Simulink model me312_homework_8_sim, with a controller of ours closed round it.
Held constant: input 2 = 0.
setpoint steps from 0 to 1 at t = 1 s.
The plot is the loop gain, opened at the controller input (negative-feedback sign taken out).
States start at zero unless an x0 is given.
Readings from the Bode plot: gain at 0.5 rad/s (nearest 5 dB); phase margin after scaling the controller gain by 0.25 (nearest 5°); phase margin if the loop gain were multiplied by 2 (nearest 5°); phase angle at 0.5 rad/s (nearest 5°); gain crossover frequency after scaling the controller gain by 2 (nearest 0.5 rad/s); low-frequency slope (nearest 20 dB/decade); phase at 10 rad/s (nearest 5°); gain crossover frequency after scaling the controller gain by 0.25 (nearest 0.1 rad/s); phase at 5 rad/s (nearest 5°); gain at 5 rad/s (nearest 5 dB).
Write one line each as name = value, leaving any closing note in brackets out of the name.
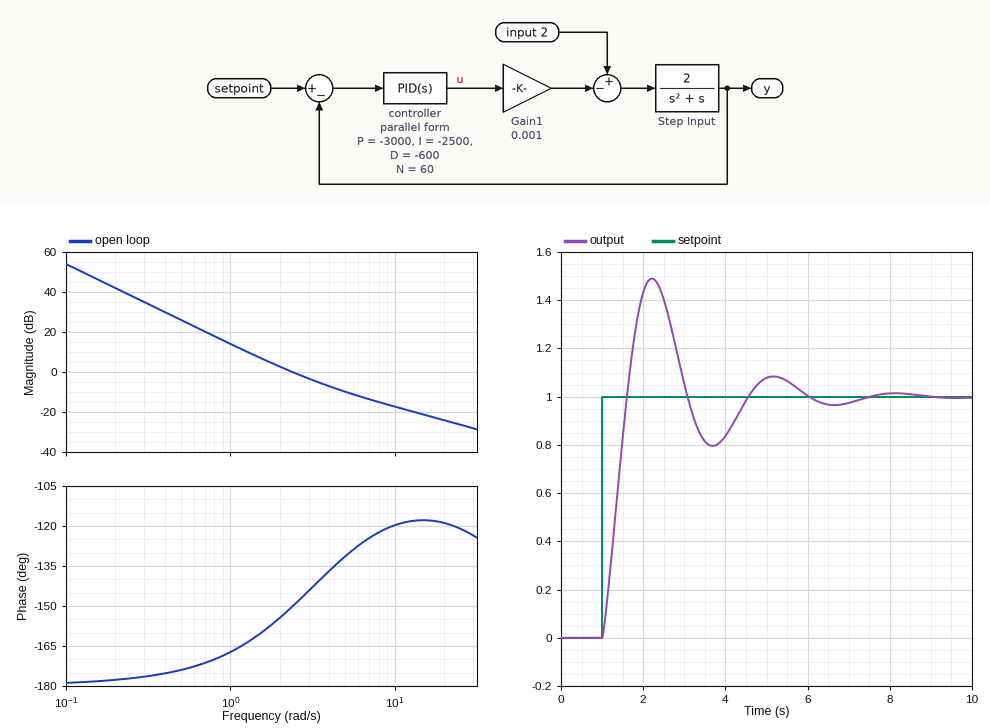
gain at 0.5 rad/s = 25 dB
phase margin after scaling the controller gain by 0.25 = 15°
phase margin if the loop gain were multiplied by 2 = 40°
phase angle at 0.5 rad/s = -175°
gain crossover frequency after scaling the controller gain by 2 = 3.5 rad/s
low-frequency slope = -40 dB/decade
phase at 10 rad/s = -120°
gain crossover frequency after scaling the controller gain by 0.25 = 1.1 rad/s
phase at 5 rad/s = -130°
gain at 5 rad/s = -10 dB
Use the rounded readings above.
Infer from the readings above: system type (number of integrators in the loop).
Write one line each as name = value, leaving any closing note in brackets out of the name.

system type = 2
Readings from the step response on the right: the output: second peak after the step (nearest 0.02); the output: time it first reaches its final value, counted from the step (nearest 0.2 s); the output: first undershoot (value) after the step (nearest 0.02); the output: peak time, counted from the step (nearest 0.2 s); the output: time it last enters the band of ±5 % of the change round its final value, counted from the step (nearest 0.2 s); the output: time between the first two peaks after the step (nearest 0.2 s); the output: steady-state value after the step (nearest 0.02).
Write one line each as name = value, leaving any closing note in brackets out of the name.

the output: second peak after the step = 1.08
the output: time it first reaches its final value, counted from the step = 0.6 s
the output: first undershoot (value) after the step = 0.80
the output: peak time, counted from the step = 1.2 s
the output: time it last enters the band of ±5 % of the change round its final value, counted from the step = 4.6 s
the output: time between the first two peaks after the step = 3.0 s
the output: steady-state value after the step = 1.00
